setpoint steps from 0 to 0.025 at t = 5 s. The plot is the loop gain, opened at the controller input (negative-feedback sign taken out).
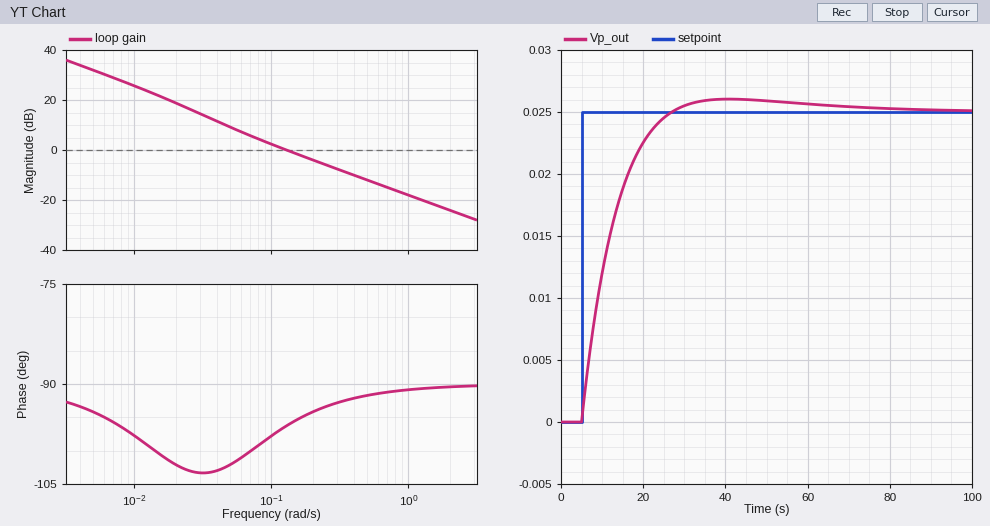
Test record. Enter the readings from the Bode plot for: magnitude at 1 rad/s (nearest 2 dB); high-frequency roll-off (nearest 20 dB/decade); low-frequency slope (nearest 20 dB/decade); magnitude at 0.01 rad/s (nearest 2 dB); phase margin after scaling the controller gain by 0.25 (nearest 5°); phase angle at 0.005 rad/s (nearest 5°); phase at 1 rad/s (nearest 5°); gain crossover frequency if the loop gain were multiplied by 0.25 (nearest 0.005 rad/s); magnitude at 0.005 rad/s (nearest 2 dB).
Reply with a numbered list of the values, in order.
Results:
1. -18 dB
2. -20 dB/decade
3. -20 dB/decade
4. 26 dB
5. 75°
6. -95°
7. -90°
8. 0.040 rad/s
9. 32 dB
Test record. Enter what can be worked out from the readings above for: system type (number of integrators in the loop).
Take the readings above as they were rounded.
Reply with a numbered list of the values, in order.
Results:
1. 1
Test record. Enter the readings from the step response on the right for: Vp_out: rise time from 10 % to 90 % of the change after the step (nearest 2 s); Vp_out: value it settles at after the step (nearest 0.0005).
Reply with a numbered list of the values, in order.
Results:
1. 14 s
2. 0.0250
